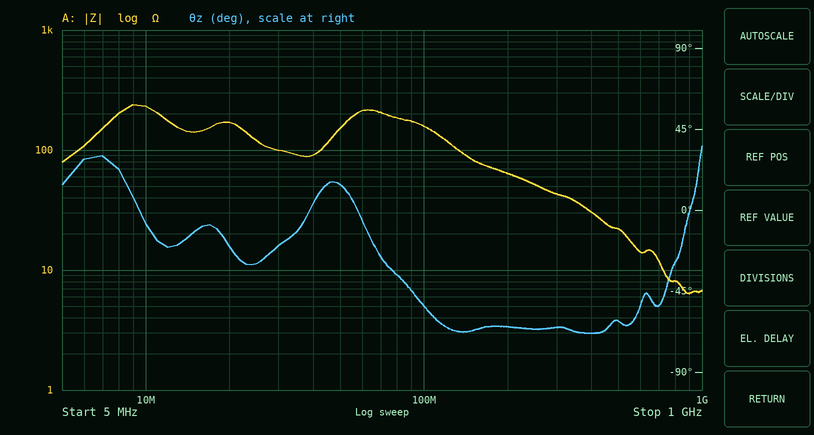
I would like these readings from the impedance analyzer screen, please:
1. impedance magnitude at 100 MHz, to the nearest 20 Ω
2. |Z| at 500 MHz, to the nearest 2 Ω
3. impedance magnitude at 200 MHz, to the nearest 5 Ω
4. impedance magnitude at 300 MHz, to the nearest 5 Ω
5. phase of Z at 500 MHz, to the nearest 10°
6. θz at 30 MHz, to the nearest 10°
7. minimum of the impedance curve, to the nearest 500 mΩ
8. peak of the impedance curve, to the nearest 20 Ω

160 Ω
22 Ω
65 Ω
45 Ω
-60°
-20°
6.5 Ω
240 Ω
